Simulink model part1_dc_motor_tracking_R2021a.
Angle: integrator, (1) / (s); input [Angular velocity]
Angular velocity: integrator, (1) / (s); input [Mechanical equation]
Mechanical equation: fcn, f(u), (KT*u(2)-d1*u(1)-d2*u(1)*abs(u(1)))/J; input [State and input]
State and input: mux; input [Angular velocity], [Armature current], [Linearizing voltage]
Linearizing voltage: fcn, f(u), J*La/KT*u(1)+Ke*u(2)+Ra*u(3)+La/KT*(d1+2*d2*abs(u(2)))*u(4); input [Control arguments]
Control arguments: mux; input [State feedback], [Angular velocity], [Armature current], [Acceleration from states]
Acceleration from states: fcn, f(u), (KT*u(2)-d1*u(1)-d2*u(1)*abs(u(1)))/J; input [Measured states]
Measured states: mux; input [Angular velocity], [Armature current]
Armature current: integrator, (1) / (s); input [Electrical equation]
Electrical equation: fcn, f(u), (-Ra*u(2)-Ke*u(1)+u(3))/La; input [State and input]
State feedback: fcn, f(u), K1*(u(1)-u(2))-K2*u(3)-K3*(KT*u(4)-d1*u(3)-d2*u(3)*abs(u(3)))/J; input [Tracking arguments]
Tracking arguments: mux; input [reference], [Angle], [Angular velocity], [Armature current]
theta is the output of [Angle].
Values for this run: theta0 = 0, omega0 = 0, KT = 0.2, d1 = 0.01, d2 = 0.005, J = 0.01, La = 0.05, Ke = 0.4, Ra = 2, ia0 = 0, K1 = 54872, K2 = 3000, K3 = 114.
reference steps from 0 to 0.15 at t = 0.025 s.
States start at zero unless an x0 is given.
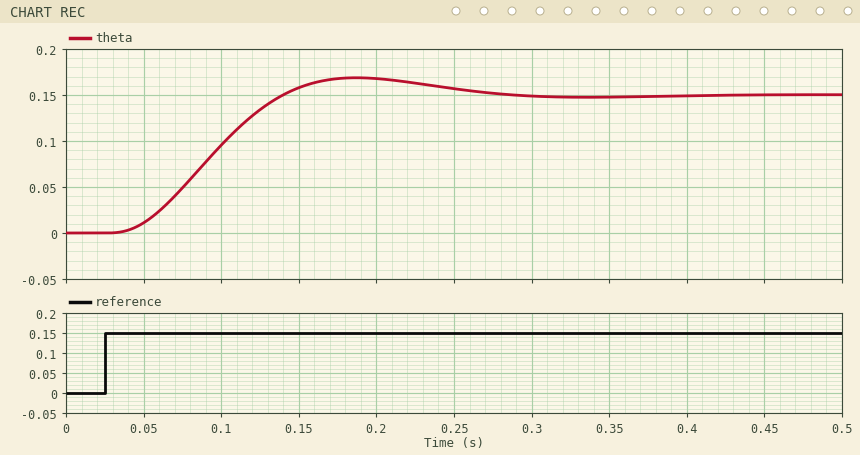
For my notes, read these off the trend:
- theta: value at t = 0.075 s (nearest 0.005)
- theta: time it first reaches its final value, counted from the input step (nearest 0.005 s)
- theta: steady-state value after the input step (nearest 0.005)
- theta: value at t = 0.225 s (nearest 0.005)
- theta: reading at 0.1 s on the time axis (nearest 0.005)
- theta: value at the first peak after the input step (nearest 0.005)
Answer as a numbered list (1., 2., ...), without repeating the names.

1. 0.050
2. 0.115 s
3. 0.150
4. 0.165
5. 0.095
6. 0.170
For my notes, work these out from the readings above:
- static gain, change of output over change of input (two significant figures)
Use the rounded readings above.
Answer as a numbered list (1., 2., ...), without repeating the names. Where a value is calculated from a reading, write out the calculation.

1. (0.15 - 0) / (0.15 - 0) = 1.0
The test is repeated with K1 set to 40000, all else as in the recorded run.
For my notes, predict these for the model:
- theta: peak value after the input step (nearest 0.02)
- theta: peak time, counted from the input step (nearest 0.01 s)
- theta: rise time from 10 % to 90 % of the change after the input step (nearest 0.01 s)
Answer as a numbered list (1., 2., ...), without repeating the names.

1. 0.16
2. 0.21 s
3. 0.10 s
